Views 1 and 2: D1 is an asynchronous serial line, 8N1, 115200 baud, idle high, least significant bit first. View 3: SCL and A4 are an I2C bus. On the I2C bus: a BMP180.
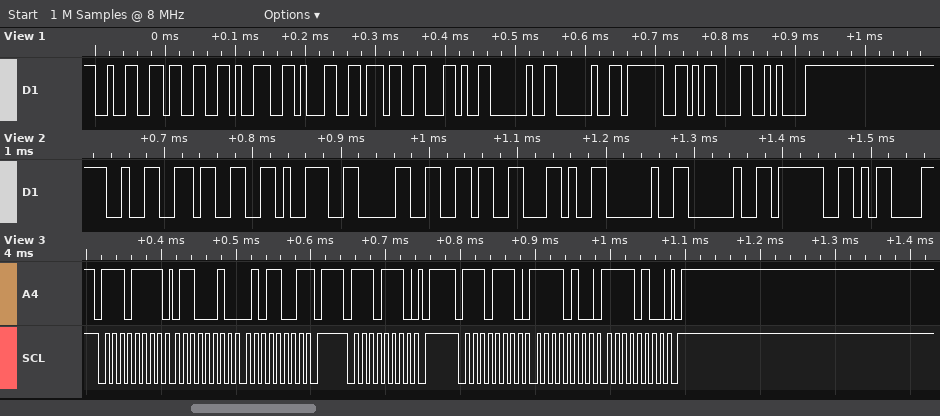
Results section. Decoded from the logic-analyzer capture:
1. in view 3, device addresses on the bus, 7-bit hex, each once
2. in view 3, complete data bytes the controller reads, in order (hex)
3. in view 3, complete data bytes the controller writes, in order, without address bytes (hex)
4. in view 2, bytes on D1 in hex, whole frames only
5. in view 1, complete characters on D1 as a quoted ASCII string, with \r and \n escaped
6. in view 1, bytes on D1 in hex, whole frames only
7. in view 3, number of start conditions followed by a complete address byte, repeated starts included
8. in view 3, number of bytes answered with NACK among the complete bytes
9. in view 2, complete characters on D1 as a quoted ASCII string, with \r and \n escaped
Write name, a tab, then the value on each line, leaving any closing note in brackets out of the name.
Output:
in view 3, device addresses on the bus, 7-bit hex, each once	0x77
in view 3, complete data bytes the controller reads, in order	62 59
in view 3, complete data bytes the controller writes, in order, without address bytes	F4 F4
in view 2, bytes on D1 in hex, whole frames only	0x32 0x33 0x39 0x30 0x36 0x2C 0x20 0x20 0x3F 0x0D
in view 1, complete characters on D1 as a quoted ASCII string, with \r and \n escaped	"23917,  ?\r\n"
in view 1, bytes on D1 in hex, whole frames only	0x32 0x33 0x39 0x31 0x37 0x2C 0x20 0x20 0x3F 0x0D 0x0A
in view 3, number of start conditions followed by a complete address byte, repeated starts included	3
in view 3, number of bytes answered with NACK among the complete bytes	1
in view 2, complete characters on D1 as a quoted ASCII string, with \r and \n escaped	"23906,  ?\r"
